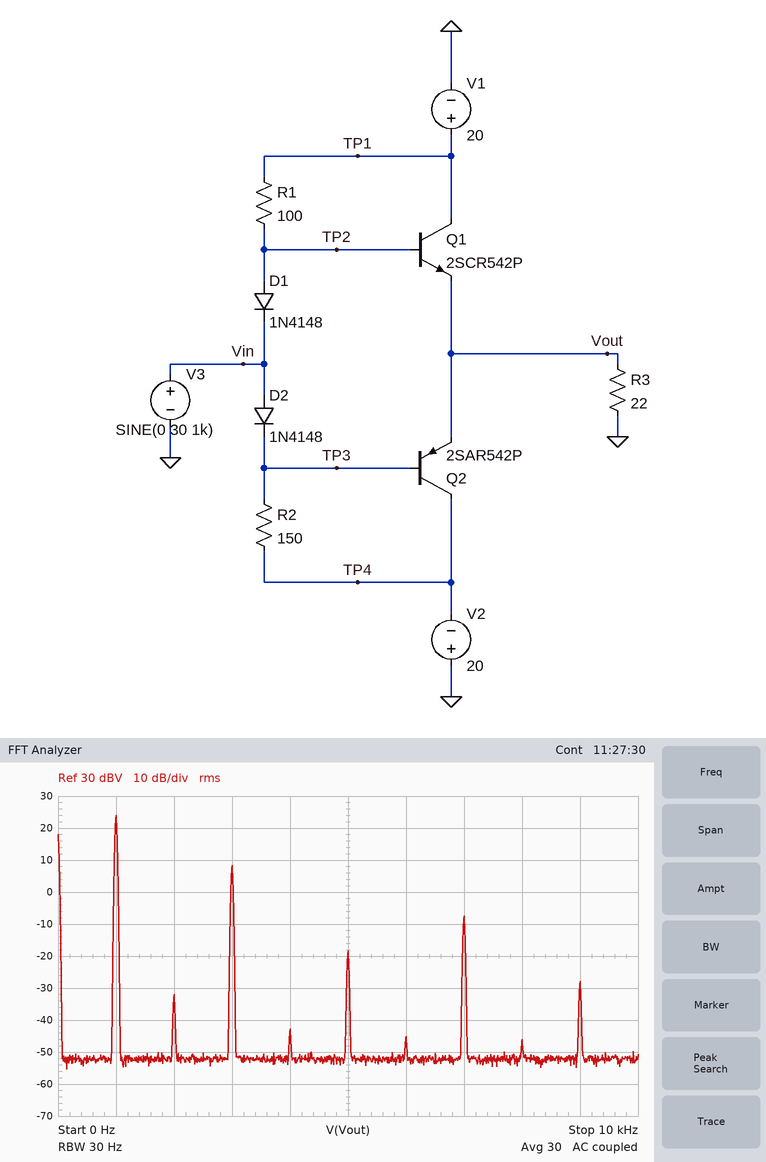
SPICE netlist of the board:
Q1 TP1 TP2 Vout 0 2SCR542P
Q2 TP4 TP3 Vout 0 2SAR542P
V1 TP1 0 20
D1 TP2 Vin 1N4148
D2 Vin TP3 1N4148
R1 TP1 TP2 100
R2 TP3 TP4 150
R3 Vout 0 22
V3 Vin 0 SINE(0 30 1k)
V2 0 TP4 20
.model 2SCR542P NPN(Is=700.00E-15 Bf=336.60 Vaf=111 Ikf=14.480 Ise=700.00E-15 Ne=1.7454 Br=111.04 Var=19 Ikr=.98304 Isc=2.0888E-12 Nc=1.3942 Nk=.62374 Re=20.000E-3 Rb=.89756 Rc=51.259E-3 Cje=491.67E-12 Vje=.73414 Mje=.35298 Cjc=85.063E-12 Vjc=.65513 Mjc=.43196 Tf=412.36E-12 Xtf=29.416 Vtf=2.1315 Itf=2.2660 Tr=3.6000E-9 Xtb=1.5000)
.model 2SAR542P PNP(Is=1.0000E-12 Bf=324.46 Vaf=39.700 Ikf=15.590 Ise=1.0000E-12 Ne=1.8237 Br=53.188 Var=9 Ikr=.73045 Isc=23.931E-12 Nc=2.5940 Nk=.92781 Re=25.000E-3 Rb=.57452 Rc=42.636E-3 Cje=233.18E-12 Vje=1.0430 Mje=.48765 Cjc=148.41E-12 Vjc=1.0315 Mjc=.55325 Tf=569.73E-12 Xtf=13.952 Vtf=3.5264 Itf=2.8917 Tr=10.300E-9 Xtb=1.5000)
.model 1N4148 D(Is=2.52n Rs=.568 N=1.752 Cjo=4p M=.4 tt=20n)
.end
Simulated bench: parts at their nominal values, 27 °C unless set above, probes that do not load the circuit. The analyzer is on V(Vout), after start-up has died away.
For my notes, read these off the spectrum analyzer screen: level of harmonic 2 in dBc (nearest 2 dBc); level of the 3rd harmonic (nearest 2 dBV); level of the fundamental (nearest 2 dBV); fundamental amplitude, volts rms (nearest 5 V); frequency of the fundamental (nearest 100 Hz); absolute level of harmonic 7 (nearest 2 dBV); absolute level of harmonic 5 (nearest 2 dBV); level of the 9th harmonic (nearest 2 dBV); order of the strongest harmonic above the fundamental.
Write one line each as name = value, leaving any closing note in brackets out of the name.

level of harmonic 2 in dBc = -56 dBc
level of the 3rd harmonic = 8 dBV
level of the fundamental = 24 dBV
fundamental amplitude, volts rms = 15 V
frequency of the fundamental = 1.0 kHz
absolute level of harmonic 7 = -8 dBV
absolute level of harmonic 5 = -18 dBV
level of the 9th harmonic = -28 dBV
order of the strongest harmonic above the fundamental = 3
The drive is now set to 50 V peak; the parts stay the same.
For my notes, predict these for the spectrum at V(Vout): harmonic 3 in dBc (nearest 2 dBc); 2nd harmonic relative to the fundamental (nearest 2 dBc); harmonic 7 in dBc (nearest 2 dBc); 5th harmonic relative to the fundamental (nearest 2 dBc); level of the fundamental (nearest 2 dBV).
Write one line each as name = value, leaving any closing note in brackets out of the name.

harmonic 3 in dBc = -12 dBc
2nd harmonic relative to the fundamental = -60 dBc
harmonic 7 in dBc = -32 dBc
5th harmonic relative to the fundamental = -20 dBc
level of the fundamental = 24 dBV
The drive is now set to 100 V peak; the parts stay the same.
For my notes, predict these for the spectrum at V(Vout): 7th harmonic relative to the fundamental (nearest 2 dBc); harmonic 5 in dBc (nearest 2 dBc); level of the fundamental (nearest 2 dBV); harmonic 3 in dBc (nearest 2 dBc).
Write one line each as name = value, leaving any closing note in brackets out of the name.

7th harmonic relative to the fundamental = -20 dBc
harmonic 5 in dBc = -16 dBc
level of the fundamental = 24 dBV
harmonic 3 in dBc = -10 dBc
